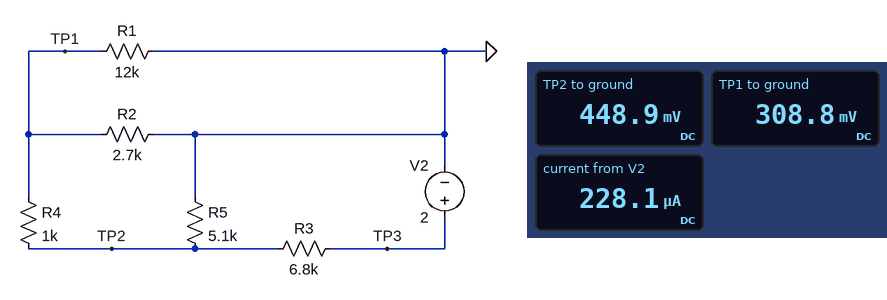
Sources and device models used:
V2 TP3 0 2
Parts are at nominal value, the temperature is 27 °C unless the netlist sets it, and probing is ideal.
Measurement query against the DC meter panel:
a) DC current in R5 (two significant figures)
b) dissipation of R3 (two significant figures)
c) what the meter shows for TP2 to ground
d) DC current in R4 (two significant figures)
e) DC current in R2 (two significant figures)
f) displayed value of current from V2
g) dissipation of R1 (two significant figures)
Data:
88 µA
350 µW
448.9 mV
140 µA
110 µA
228.1 µA
7.9 µW
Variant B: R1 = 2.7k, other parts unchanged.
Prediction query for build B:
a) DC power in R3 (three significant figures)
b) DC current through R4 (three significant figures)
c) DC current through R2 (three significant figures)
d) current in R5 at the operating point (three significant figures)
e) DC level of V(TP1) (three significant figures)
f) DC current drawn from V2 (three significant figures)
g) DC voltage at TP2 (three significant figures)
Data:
385 µW
163 µA
81.4 µA
75.0 µA
220 mV
238 µA
383 mV
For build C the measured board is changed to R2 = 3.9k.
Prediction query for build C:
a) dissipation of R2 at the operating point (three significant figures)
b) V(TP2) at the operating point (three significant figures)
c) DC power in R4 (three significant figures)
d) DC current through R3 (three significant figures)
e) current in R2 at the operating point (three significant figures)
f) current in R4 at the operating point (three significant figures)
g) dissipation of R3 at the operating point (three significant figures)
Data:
34.7 µW
493 mV
15.6 µW
222 µA
94.3 µA
125 µA
334 µW
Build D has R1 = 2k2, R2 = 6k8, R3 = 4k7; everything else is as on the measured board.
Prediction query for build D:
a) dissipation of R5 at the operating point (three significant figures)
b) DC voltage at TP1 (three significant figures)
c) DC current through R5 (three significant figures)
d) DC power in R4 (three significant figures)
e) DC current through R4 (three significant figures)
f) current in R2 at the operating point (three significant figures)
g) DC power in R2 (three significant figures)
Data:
57.7 µW
339 mV
106 µA
41.5 µW
204 µA
49.8 µA
16.9 µW
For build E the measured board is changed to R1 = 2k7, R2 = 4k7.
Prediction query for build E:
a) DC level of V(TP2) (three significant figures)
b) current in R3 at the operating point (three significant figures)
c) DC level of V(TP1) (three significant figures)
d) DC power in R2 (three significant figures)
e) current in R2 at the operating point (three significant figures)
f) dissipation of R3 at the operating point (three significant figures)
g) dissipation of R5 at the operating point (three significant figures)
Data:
413 mV
233 µA
261 mV
14.5 µW
55.6 µA
370 µW
33.5 µW
